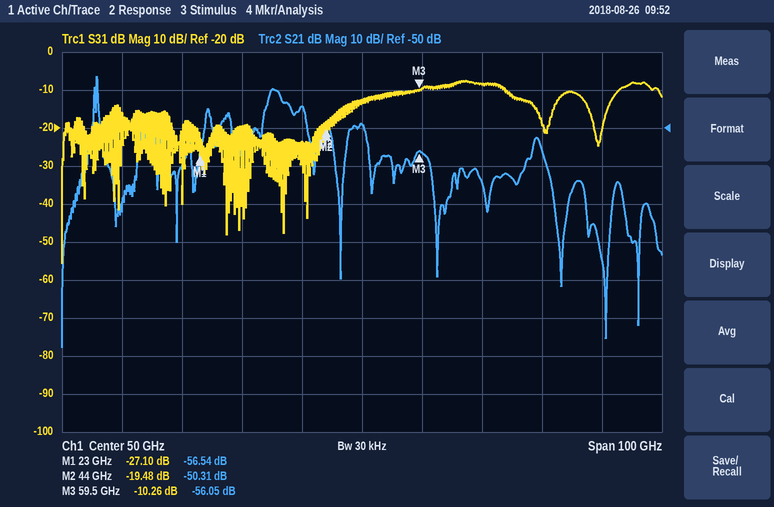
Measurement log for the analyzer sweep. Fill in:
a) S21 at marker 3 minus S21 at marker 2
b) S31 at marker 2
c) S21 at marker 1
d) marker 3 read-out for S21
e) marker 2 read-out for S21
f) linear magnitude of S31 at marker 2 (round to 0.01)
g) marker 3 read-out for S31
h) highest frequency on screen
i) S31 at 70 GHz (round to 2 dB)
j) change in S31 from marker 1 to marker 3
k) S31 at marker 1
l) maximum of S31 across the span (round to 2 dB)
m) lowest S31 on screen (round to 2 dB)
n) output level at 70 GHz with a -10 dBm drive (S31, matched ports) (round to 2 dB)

-5.74 dB
-19.48 dB
-56.54 dB
-56.05 dB
-50.31 dB
0.11
-10.26 dB
100 GHz
-8 dB
16.84 dB
-27.10 dB
-8 dB
-56 dB
-18 dBm
